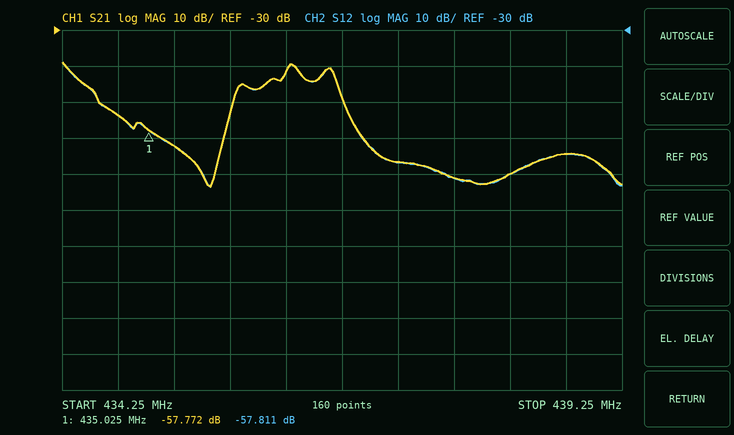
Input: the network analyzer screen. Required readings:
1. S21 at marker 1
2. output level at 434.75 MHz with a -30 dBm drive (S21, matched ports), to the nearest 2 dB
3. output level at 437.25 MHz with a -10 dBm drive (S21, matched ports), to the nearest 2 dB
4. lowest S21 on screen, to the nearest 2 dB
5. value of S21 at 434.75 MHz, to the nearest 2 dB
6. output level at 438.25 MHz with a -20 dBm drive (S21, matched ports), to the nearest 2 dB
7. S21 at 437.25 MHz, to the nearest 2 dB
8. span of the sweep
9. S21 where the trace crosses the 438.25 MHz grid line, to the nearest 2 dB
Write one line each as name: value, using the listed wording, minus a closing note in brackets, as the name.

S21 at marker 1: -57.772 dB
output level at 434.75 MHz with a -30 dBm drive (S21, matched ports), to the nearest 2 dB: -84 dBm
output level at 437.25 MHz with a -10 dBm drive (S21, matched ports), to the nearest 2 dB: -76 dBm
lowest S21 on screen, to the nearest 2 dB: -74 dB
value of S21 at 434.75 MHz, to the nearest 2 dB: -54 dB
output level at 438.25 MHz with a -20 dBm drive (S21, matched ports), to the nearest 2 dB: -90 dBm
S21 at 437.25 MHz, to the nearest 2 dB: -66 dB
span of the sweep: 5 MHz
S21 where the trace crosses the 438.25 MHz grid line, to the nearest 2 dB: -70 dB
